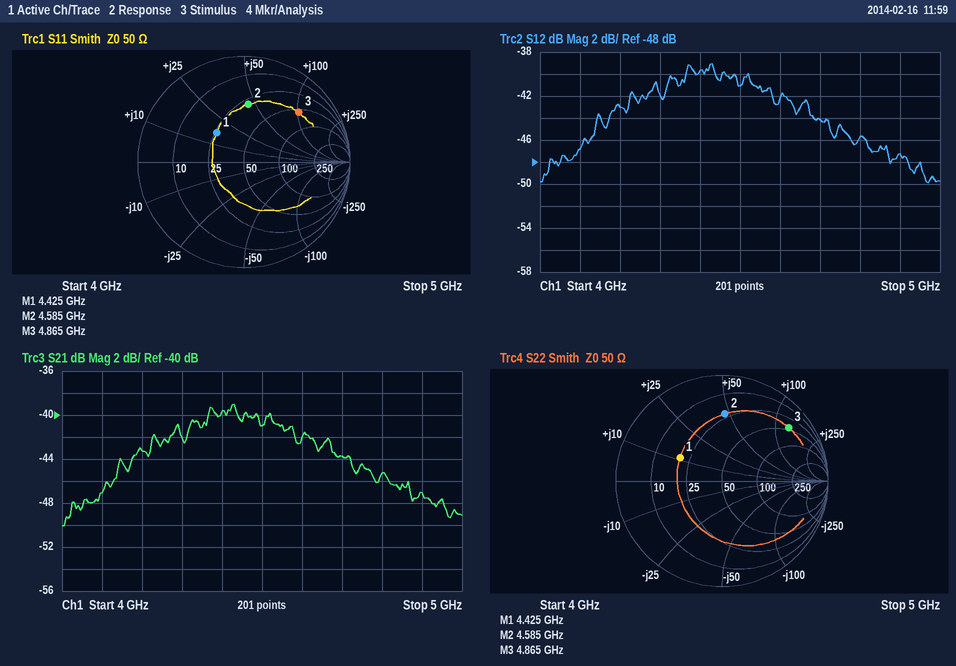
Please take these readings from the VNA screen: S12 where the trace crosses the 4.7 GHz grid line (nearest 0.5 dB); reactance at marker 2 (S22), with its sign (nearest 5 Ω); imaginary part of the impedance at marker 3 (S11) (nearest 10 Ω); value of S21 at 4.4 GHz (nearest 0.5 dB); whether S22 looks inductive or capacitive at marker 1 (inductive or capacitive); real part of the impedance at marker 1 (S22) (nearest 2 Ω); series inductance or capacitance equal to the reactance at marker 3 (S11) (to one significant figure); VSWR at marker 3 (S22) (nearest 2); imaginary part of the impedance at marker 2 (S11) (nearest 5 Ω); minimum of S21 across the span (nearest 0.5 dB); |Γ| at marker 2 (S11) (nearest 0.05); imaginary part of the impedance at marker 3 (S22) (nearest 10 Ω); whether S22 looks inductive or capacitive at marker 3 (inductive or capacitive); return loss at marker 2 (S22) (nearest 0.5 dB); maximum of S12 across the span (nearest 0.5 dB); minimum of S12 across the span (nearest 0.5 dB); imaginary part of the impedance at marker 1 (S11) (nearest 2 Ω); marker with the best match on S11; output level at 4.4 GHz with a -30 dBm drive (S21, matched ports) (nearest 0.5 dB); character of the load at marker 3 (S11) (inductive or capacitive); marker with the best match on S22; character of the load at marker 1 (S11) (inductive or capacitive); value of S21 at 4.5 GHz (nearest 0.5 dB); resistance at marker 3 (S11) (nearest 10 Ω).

-44.0 dB
+45 Ω
+100 Ω
-39.5 dB
inductive
20 Ω
3 nH
10
+45 Ω
-50.0 dB
0.55
+130 Ω
inductive
4.0 dB
-39.0 dB
-50.0 dB
+16 Ω
marker 1
-69.5 dBm
inductive
marker 1
inductive
-41.0 dB
60 Ω
